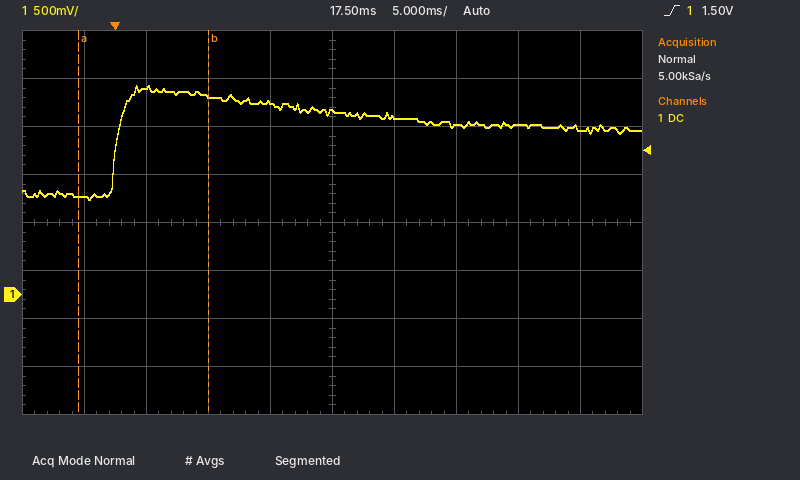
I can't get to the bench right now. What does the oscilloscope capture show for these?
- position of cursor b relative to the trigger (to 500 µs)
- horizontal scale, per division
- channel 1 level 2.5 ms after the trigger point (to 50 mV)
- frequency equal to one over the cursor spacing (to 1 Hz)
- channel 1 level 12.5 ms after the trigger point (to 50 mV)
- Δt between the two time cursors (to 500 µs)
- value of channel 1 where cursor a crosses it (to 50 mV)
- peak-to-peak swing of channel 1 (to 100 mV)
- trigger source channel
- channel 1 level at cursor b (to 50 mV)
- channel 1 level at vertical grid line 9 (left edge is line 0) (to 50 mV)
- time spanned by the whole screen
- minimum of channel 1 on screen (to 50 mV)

+7.5 ms
5 ms
2.15 V
95 Hz
2.00 V
10.5 ms
1.00 V
1.20 V
channel 1
2.05 V
1.70 V
50 ms
1.00 V
